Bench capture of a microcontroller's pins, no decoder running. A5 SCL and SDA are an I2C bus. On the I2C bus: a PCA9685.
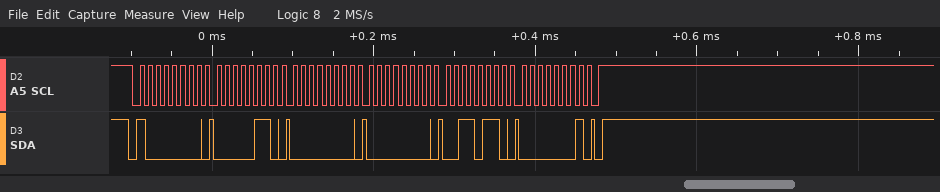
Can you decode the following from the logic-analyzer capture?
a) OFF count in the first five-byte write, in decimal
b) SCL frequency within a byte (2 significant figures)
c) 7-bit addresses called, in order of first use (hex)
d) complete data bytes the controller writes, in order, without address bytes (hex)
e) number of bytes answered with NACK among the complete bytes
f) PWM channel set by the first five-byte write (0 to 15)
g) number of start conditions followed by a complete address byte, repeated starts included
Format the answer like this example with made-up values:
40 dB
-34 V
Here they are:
310
100 kHz
0x40
06 00 00 36 01
0
0
1
